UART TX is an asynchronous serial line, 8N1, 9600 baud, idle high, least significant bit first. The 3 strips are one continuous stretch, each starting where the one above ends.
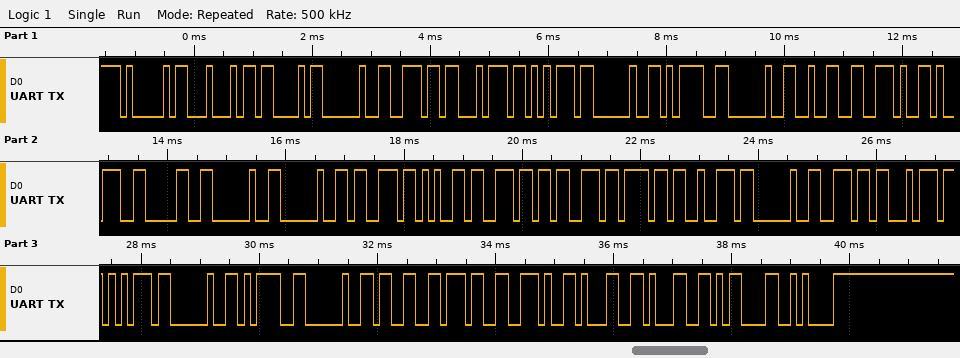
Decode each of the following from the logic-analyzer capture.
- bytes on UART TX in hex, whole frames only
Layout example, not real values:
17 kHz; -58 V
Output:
0x41 0x44 0x43 0x20 0x6E 0x74 0x75 0x20 0x3D 0x20 0x32 0x2E 0x39 0x30 0x20 0x20 0x73 0x65 0x6E 0x73 0x6F 0x72 0x20 0x6E 0x74 0x75 0x20 0x3D 0x20 0x33 0x37 0x2E 0x31 0x31 0x0D 0x0A
